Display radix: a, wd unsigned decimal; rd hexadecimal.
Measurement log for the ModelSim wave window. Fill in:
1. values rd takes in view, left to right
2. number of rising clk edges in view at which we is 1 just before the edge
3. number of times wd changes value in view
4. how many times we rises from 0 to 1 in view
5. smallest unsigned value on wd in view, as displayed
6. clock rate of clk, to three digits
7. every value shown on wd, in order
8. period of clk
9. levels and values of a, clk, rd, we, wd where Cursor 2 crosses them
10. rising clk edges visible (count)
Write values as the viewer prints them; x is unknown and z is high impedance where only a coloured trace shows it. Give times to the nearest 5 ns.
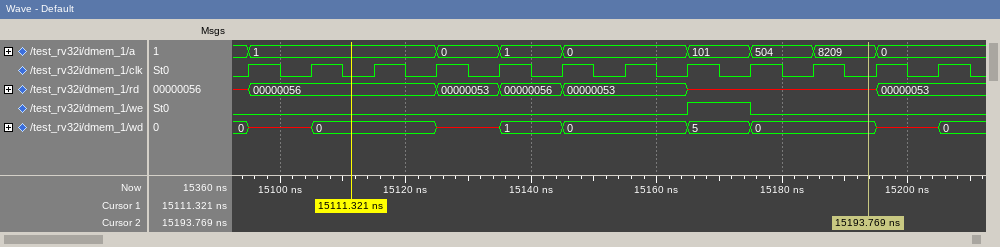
x, 00000056, 00000053, 00000056, 00000053, x, 00000053
1
9
1
0
100 MHz
0, x, 0, x, 1, 0, 5, 0, x, 0
10 ns
a=8209, clk=0, rd=x, we=0, wd=0
12
